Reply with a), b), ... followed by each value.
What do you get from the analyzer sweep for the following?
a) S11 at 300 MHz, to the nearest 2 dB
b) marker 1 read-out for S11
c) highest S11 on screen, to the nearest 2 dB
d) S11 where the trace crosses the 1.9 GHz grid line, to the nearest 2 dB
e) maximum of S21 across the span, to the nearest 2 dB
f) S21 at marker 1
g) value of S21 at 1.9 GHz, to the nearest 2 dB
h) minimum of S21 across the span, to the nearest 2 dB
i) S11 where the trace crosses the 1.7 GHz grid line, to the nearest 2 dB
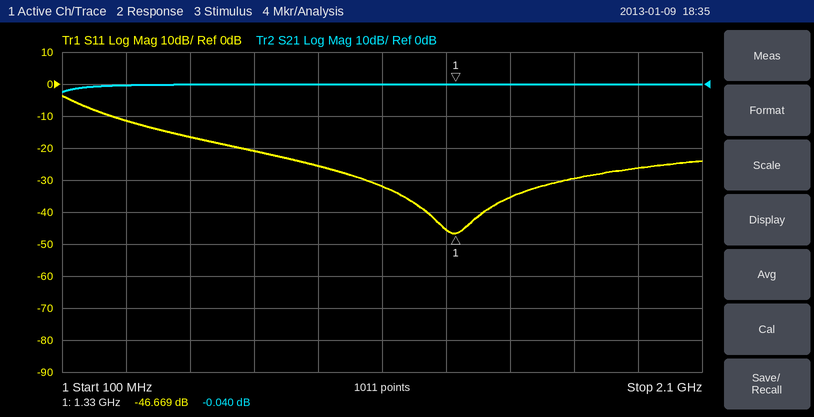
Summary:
a) -12 dB
b) -46.669 dB
c) -4 dB
d) -26 dB
e) 0 dB
f) -0.040 dB
g) 0 dB
h) -2 dB
i) -30 dB
